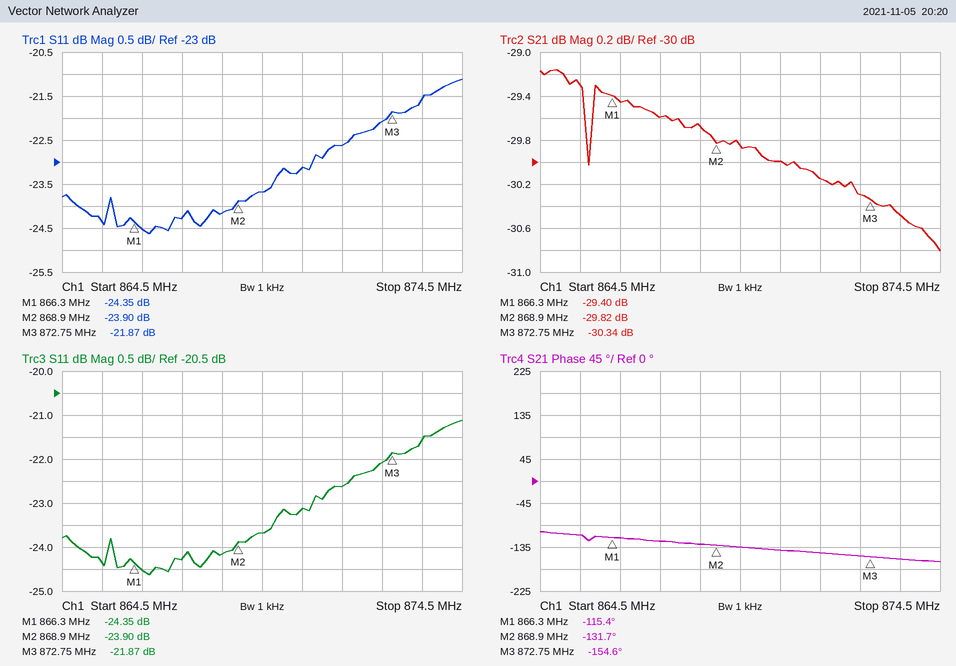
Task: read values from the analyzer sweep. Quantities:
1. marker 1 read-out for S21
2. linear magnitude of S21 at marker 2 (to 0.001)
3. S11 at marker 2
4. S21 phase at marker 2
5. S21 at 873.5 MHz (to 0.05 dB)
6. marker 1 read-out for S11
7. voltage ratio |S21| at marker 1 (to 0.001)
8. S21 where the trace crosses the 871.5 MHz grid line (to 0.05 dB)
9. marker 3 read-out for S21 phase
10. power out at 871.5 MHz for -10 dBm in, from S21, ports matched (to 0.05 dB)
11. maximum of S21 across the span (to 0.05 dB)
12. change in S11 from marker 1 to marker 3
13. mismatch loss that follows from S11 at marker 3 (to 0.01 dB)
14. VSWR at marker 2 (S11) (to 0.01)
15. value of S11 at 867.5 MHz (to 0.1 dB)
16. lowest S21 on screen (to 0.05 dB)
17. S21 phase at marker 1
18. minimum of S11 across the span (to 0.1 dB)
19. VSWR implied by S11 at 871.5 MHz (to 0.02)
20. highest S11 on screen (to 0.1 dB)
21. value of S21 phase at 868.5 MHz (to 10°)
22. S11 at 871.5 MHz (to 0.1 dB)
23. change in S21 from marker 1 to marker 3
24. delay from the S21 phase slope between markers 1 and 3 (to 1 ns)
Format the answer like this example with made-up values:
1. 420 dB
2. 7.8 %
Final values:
1. -29.40 dB
2. 0.032
3. -23.90 dB
4. -131.7°
5. -30.50 dB
6. -24.35 dB
7. 0.034
8. -30.15 dB
9. -154.6°
10. -40.15 dBm
11. -29.15 dB
12. 2.48 dB
13. 0.03 dB
14. 1.14
15. -24.3 dB
16. -30.80 dB
17. -115.4°
18. -24.6 dB
19. 1.16
20. -21.1 dB
21. -130°
22. -22.6 dB
23. -0.94 dB
24. 17 ns
